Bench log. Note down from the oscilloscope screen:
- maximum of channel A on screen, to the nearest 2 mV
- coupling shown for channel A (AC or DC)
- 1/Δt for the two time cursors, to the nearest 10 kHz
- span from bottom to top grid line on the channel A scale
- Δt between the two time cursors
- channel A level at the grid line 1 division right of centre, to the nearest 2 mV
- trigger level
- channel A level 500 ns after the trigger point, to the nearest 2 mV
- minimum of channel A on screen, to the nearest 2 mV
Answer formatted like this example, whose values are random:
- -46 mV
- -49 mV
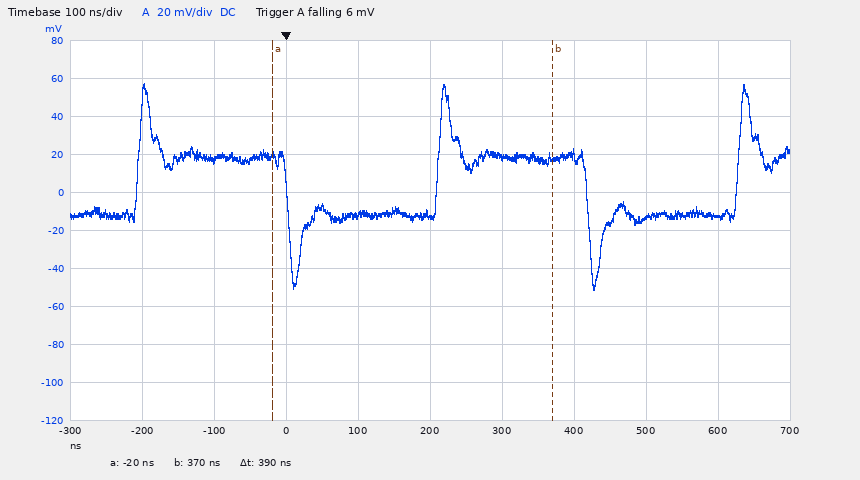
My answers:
- 58 mV
- DC
- 2.56 MHz
- 200 mV
- 390 ns
- 18 mV
- 6 mV
- -12 mV
- -52 mV
